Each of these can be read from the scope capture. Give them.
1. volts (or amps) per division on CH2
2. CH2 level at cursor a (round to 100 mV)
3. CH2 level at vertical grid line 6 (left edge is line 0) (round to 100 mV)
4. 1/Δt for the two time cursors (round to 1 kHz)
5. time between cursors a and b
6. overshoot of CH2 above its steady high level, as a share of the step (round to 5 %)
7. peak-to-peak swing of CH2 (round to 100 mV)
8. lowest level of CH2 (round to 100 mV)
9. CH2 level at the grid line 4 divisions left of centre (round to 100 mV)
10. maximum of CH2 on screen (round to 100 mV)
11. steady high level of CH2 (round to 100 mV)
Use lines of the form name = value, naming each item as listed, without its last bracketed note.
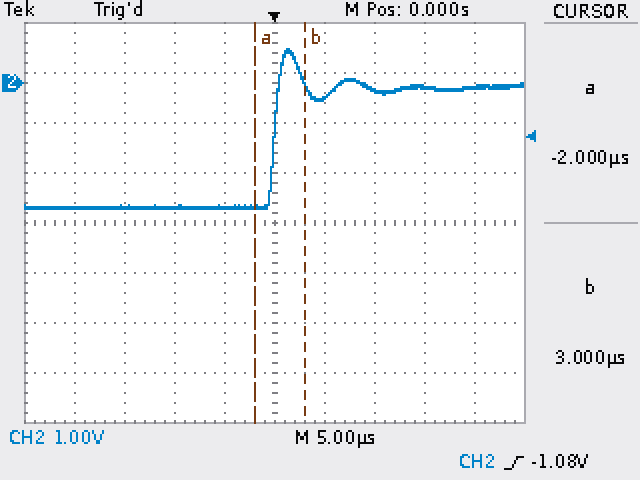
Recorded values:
volts (or amps) per division on CH2 = 1 V
CH2 level at cursor a = -2.5 V
CH2 level at vertical grid line 6 (left edge is line 0) = -300 mV
1/Δt for the two time cursors = 200 kHz
time between cursors a and b = 5.0 µs
overshoot of CH2 above its steady high level, as a share of the step = 30 %
peak-to-peak swing of CH2 = 3.2 V
lowest level of CH2 = -2.5 V
CH2 level at the grid line 4 divisions left of centre = -2.5 V
maximum of CH2 on screen = 700 mV
steady high level of CH2 = -100 mV
